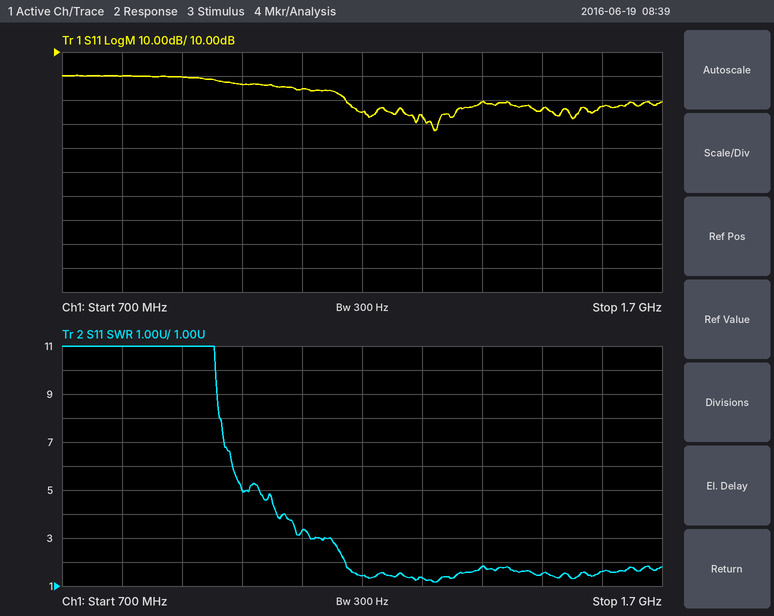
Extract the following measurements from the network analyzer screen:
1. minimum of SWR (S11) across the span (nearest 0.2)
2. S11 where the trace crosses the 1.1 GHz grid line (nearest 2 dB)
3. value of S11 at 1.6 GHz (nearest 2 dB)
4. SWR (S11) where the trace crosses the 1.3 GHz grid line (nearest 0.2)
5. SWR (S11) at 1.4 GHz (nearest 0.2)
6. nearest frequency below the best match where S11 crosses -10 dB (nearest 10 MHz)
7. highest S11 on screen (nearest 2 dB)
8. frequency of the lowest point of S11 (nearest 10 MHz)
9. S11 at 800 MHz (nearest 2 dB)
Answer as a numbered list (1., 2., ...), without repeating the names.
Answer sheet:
1. 1.2
2. -6 dB
3. -12 dB
4. 1.4
5. 1.8
6. 1.17 GHz
7. 0 dB
8. 1.32 GHz
9. 0 dB
